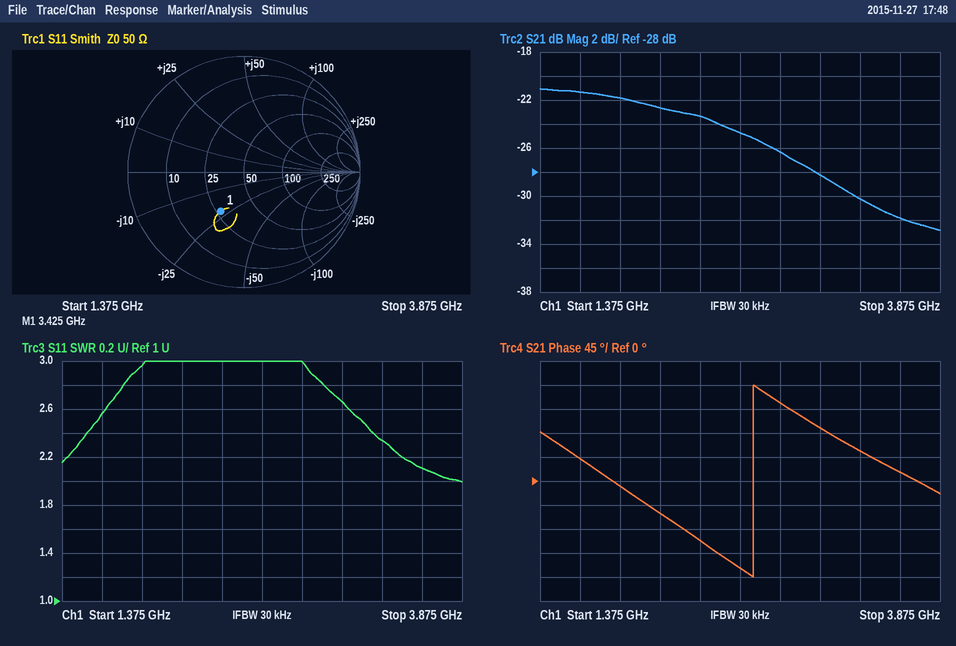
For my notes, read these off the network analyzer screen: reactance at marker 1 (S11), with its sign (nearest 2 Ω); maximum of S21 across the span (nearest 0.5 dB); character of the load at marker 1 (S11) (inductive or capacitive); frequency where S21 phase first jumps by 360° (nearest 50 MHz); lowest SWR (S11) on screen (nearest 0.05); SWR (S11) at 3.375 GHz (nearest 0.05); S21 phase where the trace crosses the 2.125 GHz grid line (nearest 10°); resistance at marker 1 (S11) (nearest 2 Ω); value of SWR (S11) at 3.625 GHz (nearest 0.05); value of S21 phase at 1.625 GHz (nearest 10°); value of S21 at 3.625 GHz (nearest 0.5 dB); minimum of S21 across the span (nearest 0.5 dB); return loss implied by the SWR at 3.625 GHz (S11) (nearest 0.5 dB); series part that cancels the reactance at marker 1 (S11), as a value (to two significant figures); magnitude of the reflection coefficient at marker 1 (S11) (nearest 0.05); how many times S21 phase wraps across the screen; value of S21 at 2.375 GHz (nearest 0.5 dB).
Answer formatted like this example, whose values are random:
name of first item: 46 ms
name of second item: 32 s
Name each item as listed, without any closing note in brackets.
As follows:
reactance at marker 1 (S11), with its sign: -22 Ω
maximum of S21 across the span: -21.0 dB
character of the load at marker 1 (S11): capacitive
frequency where S21 phase first jumps by 360°: 2.70 GHz
lowest SWR (S11) on screen: 2.00
SWR (S11) at 3.375 GHz: 2.35
S21 phase where the trace crosses the 2.125 GHz grid line: -60°
resistance at marker 1 (S11): 28 Ω
value of SWR (S11) at 3.625 GHz: 2.10
value of S21 phase at 1.625 GHz: 40°
value of S21 at 3.625 GHz: -32.0 dB
minimum of S21 across the span: -33.0 dB
return loss implied by the SWR at 3.625 GHz (S11): 9.0 dB
series part that cancels the reactance at marker 1 (S11), as a value: 1.0 nH
magnitude of the reflection coefficient at marker 1 (S11): 0.40
how many times S21 phase wraps across the screen: 1
value of S21 at 2.375 GHz: -23.5 dB
